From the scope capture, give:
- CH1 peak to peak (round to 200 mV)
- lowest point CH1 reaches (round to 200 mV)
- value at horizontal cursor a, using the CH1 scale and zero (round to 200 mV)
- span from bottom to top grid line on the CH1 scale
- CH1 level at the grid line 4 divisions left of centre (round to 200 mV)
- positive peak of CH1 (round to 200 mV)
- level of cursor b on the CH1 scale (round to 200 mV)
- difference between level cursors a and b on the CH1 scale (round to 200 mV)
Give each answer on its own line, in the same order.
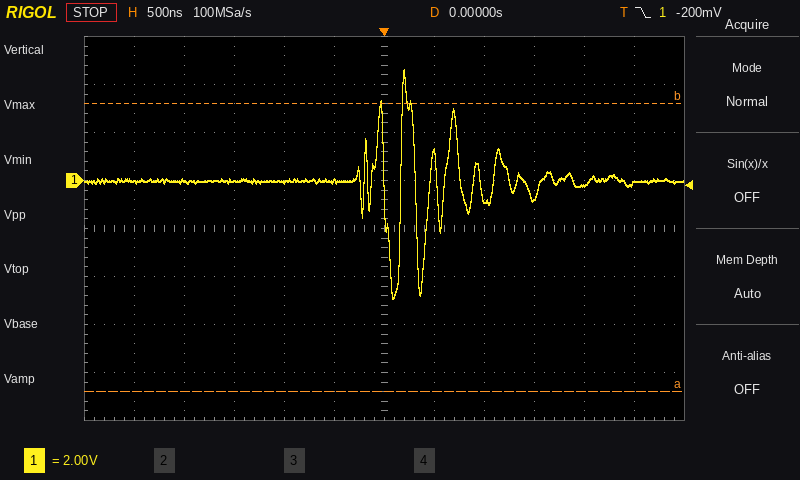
9.6 V
-5.0 V
-8.8 V
16 V
0.0 V
4.6 V
3.2 V
12.0 V
